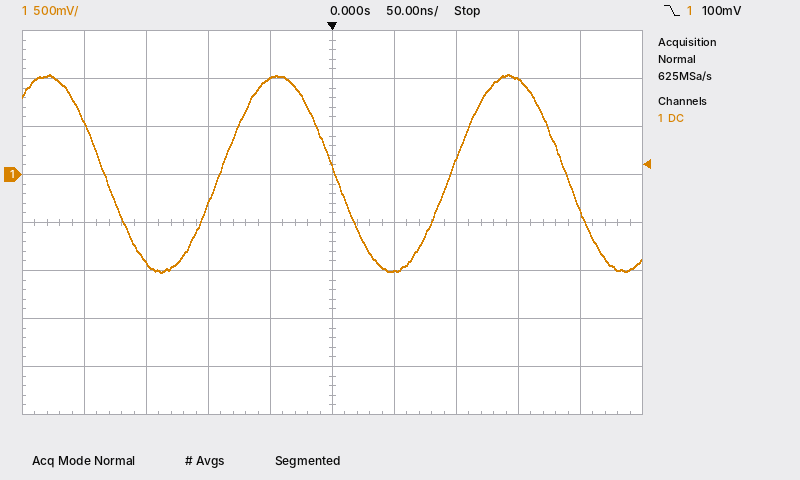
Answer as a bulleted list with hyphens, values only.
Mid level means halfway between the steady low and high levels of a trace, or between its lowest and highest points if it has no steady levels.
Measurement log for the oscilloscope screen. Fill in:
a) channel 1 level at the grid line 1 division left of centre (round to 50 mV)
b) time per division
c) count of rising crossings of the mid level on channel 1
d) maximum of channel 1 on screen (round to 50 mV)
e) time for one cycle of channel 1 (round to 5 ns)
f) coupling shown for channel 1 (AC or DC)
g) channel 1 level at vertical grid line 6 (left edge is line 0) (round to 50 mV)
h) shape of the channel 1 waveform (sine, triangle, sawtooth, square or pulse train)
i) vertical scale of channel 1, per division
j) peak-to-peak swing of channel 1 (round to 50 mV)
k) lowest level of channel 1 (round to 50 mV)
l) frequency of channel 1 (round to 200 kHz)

- 1.00 V
- 50 ns
- 2
- 1.05 V
- 185 ns
- DC
- -1.00 V
- sine
- 500 mV
- 2.05 V
- -1.00 V
- 5.4 MHz
